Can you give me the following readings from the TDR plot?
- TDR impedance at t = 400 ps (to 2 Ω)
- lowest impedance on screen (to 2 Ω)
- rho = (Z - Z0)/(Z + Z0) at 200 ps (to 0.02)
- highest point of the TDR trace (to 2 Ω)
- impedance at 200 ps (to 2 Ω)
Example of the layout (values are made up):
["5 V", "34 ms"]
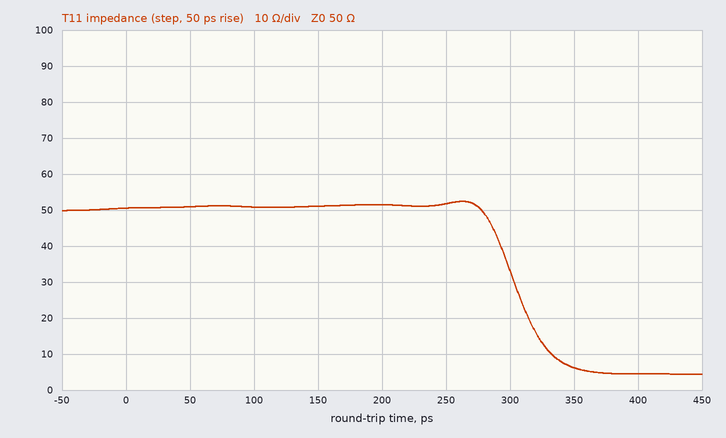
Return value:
["4 Ω", "4 Ω", "+0.02", "52 Ω", "52 Ω"]
